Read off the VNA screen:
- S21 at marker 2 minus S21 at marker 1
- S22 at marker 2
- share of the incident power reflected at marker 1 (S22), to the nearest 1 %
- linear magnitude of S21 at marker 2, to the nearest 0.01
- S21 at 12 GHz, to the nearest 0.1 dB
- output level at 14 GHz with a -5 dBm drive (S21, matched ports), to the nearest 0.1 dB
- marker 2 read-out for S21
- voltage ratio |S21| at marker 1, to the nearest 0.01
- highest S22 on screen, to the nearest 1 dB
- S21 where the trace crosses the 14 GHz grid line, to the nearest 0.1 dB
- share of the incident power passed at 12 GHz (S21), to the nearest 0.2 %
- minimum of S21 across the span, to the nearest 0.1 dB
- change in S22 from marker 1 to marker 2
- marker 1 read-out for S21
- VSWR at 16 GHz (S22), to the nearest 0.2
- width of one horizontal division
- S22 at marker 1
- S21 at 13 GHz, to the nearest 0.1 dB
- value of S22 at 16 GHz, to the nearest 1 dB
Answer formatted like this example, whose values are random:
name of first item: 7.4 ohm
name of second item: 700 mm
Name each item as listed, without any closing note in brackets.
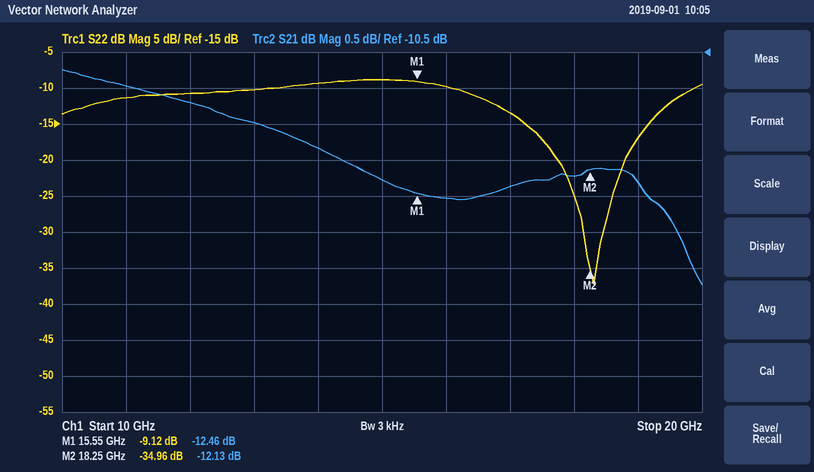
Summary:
S21 at marker 2 minus S21 at marker 1: 0.33 dB
S22 at marker 2: -34.96 dB
share of the incident power reflected at marker 1 (S22), to the nearest 1 %: 12 %
linear magnitude of S21 at marker 2, to the nearest 0.01: 0.25
S21 at 12 GHz, to the nearest 0.1 dB: -11.2 dB
output level at 14 GHz with a -5 dBm drive (S21, matched ports), to the nearest 0.1 dB: -16.8 dBm
marker 2 read-out for S21: -12.13 dB
voltage ratio |S21| at marker 1, to the nearest 0.01: 0.24
highest S22 on screen, to the nearest 1 dB: -9 dB
S21 where the trace crosses the 14 GHz grid line, to the nearest 0.1 dB: -11.8 dB
share of the incident power passed at 12 GHz (S21), to the nearest 0.2 %: 7.6 %
minimum of S21 across the span, to the nearest 0.1 dB: -13.7 dB
change in S22 from marker 1 to marker 2: -25.84 dB
marker 1 read-out for S21: -12.46 dB
VSWR at 16 GHz (S22), to the nearest 0.2: 2.0
width of one horizontal division: 1 GHz
S22 at marker 1: -9.12 dB
S21 at 13 GHz, to the nearest 0.1 dB: -11.5 dB
value of S22 at 16 GHz, to the nearest 1 dB: -10 dB
